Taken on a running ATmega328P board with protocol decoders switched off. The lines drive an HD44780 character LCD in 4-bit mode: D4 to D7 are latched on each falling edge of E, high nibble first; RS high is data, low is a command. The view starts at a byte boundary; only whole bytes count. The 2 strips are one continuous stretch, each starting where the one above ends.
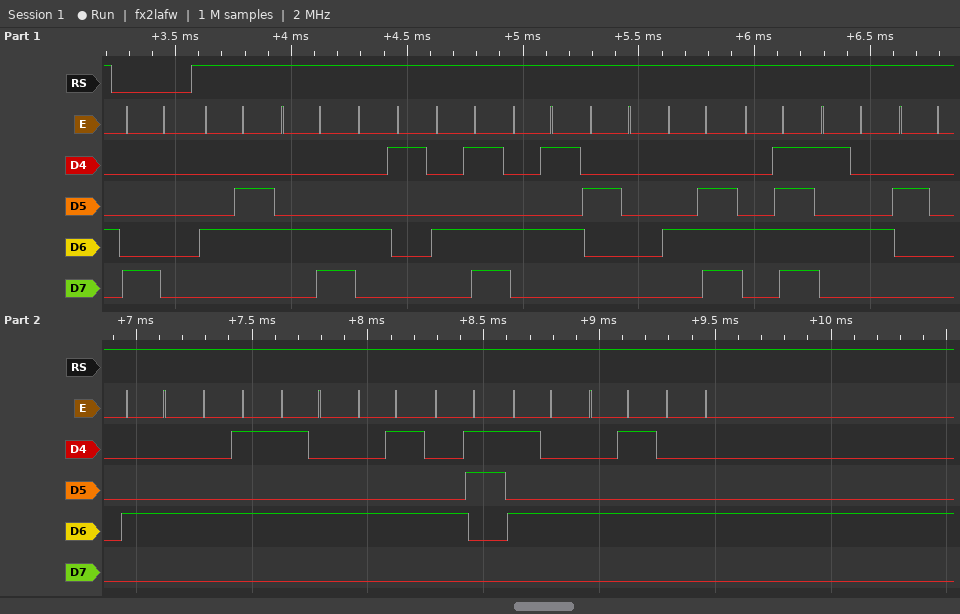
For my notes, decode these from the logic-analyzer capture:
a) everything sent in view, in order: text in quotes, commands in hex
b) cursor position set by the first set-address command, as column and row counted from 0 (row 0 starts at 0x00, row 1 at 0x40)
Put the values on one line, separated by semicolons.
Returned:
0x80 "FLAME NOT DETECTED"; column 0, row 0
